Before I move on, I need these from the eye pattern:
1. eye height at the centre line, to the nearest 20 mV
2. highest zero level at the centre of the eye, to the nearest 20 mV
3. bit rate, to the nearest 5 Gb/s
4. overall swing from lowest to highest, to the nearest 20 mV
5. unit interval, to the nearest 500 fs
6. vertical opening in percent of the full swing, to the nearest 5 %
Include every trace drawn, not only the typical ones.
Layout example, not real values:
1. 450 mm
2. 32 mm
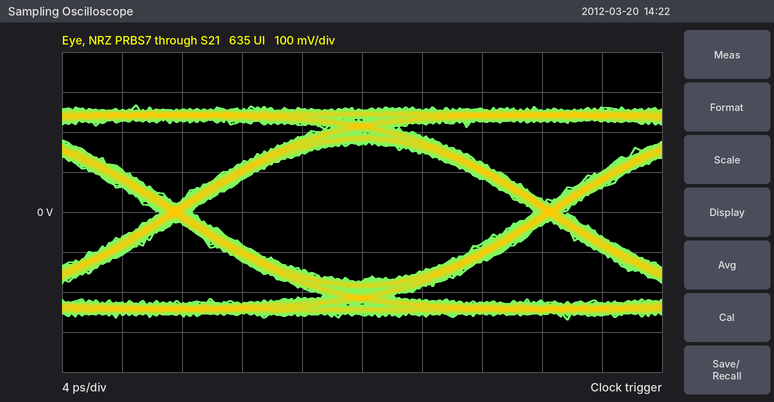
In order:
1. 340 mV
2. -180 mV
3. 40 Gb/s
4. 540 mV
5. 25.0 ps
6. 65 %
